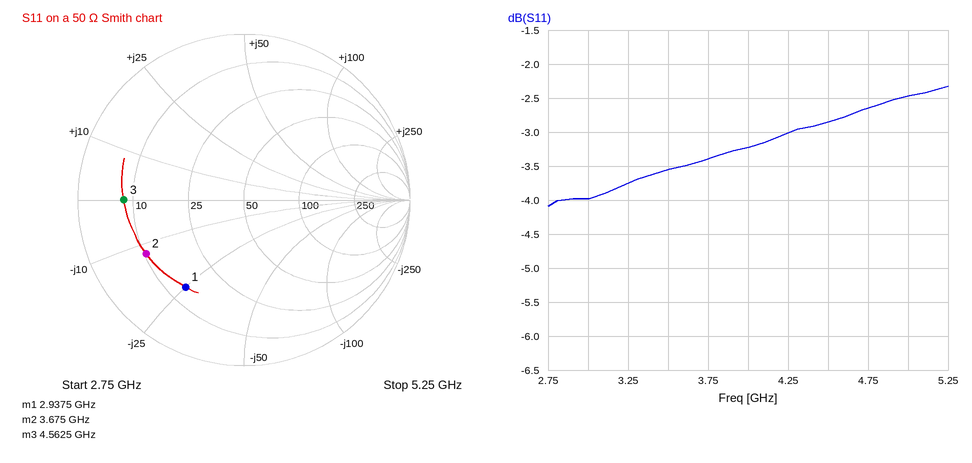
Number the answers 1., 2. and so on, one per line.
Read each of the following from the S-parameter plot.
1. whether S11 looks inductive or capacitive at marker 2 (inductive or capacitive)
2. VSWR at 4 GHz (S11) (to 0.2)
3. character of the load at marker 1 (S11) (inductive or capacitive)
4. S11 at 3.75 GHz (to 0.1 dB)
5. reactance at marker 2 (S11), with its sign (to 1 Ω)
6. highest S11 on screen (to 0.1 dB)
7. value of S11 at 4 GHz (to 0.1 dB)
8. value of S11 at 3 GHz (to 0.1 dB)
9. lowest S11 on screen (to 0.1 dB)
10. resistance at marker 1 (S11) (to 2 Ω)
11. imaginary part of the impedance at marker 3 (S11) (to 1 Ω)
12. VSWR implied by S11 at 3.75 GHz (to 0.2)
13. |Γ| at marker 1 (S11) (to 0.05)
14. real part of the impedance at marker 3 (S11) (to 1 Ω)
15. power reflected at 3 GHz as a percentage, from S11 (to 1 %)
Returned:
1. capacitive
2. 5.4
3. capacitive
4. -3.4 dB
5. -12 Ω
6. -2.3 dB
7. -3.2 dB
8. -4.0 dB
9. -4.1 dB
10. 14 Ω
11. 0 Ω
12. 5.2
13. 0.65
14. 8 Ω
15. 40 %
